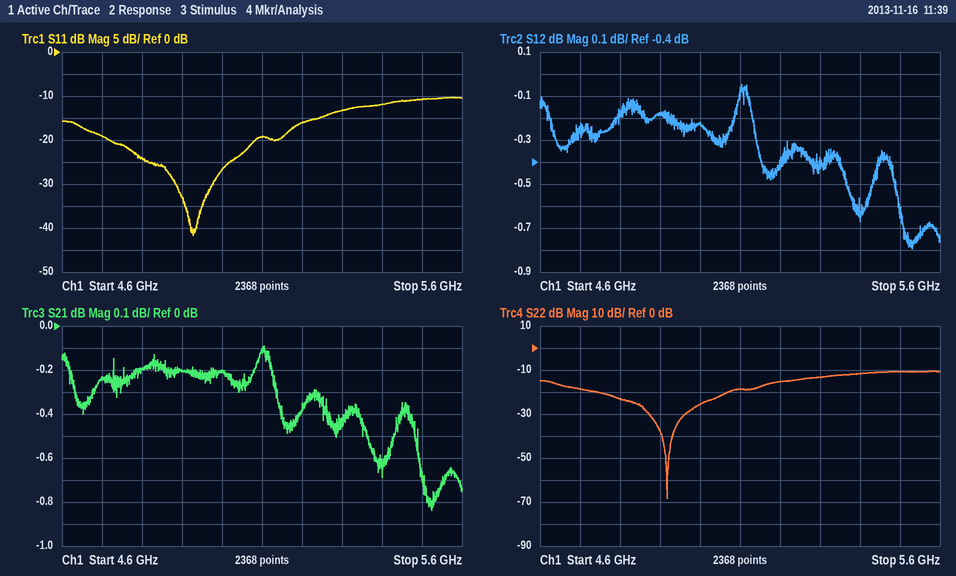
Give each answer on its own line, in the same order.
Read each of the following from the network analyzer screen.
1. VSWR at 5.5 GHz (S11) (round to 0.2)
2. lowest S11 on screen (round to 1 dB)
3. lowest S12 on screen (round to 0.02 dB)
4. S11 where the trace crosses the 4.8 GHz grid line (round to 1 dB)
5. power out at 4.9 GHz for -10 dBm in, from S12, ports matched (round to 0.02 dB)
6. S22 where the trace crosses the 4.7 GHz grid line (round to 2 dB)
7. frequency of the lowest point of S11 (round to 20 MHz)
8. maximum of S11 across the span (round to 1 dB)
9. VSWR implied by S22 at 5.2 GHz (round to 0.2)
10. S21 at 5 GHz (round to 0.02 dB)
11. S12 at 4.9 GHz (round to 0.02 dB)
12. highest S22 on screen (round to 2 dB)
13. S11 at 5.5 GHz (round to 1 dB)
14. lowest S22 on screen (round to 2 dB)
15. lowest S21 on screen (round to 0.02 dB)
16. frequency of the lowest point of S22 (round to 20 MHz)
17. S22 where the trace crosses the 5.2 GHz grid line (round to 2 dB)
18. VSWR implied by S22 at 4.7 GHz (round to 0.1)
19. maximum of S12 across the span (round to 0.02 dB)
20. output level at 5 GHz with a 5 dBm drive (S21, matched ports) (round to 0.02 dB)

1.8
-42 dB
-0.80 dB
-24 dB
-10.18 dBm
-18 dB
4.92 GHz
-10 dB
1.4
-0.20 dB
-0.18 dB
-10 dB
-11 dB
-68 dB
-0.84 dB
4.92 GHz
-16 dB
1.3
-0.04 dB
4.80 dBm
